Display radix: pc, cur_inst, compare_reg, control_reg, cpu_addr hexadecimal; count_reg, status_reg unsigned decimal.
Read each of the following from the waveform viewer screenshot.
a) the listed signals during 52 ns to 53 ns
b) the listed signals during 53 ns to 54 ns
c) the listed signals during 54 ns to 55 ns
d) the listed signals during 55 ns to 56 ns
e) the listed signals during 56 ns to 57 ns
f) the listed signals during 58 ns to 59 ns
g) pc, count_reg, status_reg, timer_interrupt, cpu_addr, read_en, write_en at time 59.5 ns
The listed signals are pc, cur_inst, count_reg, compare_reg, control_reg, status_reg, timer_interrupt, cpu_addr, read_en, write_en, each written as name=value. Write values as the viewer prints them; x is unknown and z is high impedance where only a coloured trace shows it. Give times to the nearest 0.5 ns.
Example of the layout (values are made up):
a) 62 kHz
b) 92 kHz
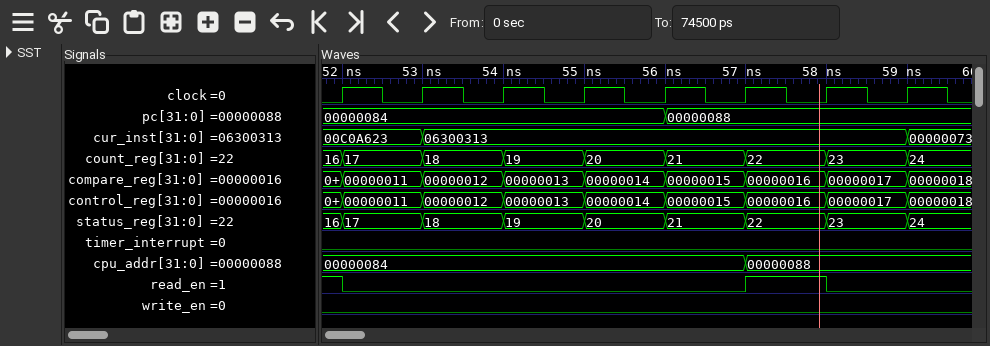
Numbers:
a) pc=00000084, cur_inst=00C0A623, count_reg=17, compare_reg=00000011, control_reg=00000011, status_reg=17, timer_interrupt=0, cpu_addr=00000084, read_en=0, write_en=0
b) pc=00000084, cur_inst=06300313, count_reg=18, compare_reg=00000012, control_reg=00000012, status_reg=18, timer_interrupt=0, cpu_addr=00000084, read_en=0, write_en=0
c) pc=00000084, cur_inst=06300313, count_reg=19, compare_reg=00000013, control_reg=00000013, status_reg=19, timer_interrupt=0, cpu_addr=00000084, read_en=0, write_en=0
d) pc=00000084, cur_inst=06300313, count_reg=20, compare_reg=00000014, control_reg=00000014, status_reg=20, timer_interrupt=0, cpu_addr=00000084, read_en=0, write_en=0
e) pc=00000088, cur_inst=06300313, count_reg=21, compare_reg=00000015, control_reg=00000015, status_reg=21, timer_interrupt=0, cpu_addr=00000084, read_en=0, write_en=0
f) pc=00000088, cur_inst=06300313, count_reg=23, compare_reg=00000017, control_reg=00000017, status_reg=23, timer_interrupt=0, cpu_addr=00000088, read_en=0, write_en=0
g) pc=00000088, count_reg=24, status_reg=24, timer_interrupt=0, cpu_addr=00000088, read_en=0, write_en=0
